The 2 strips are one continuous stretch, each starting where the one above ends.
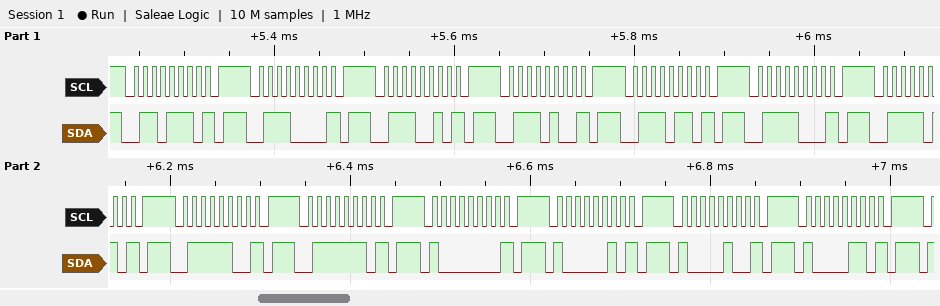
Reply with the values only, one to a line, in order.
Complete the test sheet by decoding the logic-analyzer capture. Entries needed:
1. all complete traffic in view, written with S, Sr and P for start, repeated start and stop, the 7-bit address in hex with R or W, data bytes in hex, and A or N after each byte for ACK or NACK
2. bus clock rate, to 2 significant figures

S 37W N P S 38W N P S 39W N P S 3AW N P S 3BW N P S 3CW N P S 3DW N P S 3EW N P S 3FW N P S 40W N P S 41W N P S 42W N P S 43W N P
100 kHz
